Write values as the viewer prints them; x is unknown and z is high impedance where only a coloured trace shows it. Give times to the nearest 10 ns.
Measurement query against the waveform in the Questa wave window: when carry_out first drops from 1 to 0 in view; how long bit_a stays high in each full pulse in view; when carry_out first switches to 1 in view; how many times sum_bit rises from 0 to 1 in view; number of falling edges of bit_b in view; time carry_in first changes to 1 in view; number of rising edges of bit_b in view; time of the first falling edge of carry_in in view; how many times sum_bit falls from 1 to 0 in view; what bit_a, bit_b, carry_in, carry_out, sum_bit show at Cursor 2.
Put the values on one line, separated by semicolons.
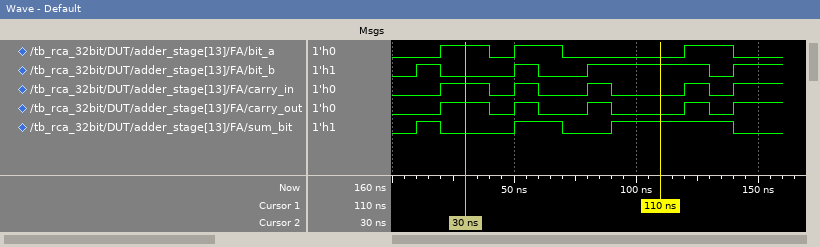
40 ns; 20 ns, 20 ns, 20 ns; 20 ns; 3; 3; 20 ns; 4; 40 ns; 3; bit_a=1, bit_b=0, carry_in=1, carry_out=1, sum_bit=0
